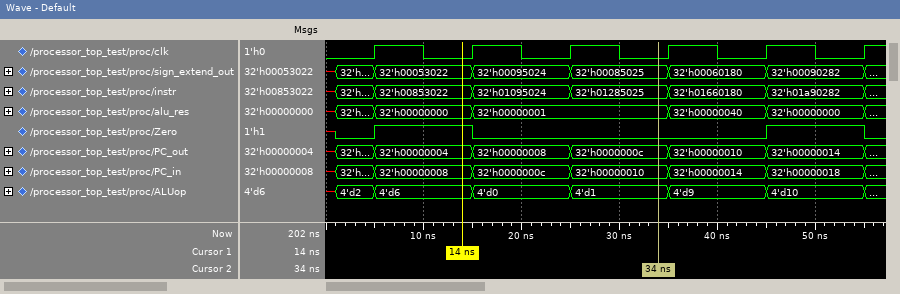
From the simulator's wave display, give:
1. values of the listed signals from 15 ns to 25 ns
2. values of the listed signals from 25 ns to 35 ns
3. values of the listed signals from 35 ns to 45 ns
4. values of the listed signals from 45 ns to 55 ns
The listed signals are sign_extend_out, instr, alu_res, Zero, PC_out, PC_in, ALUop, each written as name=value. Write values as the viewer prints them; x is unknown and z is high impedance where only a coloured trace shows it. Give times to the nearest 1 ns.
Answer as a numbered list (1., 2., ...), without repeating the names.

1. sign_extend_out=32'h00095024, instr=32'h01095024, alu_res=32'h00000001, Zero=0, PC_out=32'h00000008, PC_in=32'h0000000c, ALUop=4'd0
2. sign_extend_out=32'h00085025, instr=32'h01285025, alu_res=32'h00000001, Zero=0, PC_out=32'h0000000c, PC_in=32'h00000010, ALUop=4'd1
3. sign_extend_out=32'h00060180, instr=32'h01660180, alu_res=32'h00000040, Zero=0, PC_out=32'h00000010, PC_in=32'h00000014, ALUop=4'd9
4. sign_extend_out=32'h00090282, instr=32'h01a90282, alu_res=32'h00000000, Zero=1, PC_out=32'h00000014, PC_in=32'h00000018, ALUop=4'd10
